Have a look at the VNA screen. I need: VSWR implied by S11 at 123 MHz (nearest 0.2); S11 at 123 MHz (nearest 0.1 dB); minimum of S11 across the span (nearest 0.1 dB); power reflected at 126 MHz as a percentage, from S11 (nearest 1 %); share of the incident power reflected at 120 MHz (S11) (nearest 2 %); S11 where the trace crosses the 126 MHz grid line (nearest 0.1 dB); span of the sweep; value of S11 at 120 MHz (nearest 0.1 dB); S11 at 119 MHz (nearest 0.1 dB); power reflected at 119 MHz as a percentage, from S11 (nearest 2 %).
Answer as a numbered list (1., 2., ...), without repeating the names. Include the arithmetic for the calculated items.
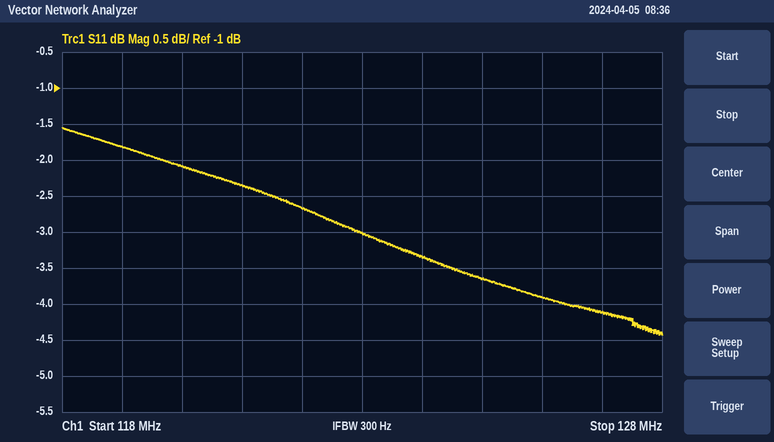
1. |Γ| = 10^(-3/20) = 0.7079; VSWR = (1 + 0.7079)/(1 − 0.7079) ≈ 5.8
2. -3.0 dB
3. -4.4 dB
4. 10^(-3.9/10) ≈ 41 %
5. 10^(-2.1/10) ≈ 62 %
6. -3.9 dB
7. 10 MHz
8. -2.1 dB
9. -1.8 dB
10. 10^(-1.8/10) ≈ 66 %
